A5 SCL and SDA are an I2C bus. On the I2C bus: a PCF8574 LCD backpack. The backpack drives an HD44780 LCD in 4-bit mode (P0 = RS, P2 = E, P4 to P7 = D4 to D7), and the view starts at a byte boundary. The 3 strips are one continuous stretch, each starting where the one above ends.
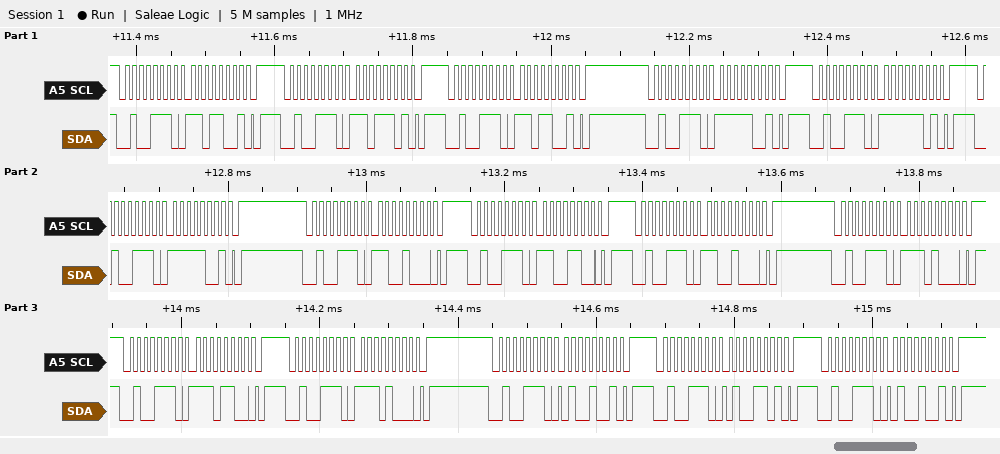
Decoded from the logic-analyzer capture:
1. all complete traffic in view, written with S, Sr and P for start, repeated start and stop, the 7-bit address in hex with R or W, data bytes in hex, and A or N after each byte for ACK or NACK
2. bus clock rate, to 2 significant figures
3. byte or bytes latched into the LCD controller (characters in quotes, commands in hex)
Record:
S 27W A D9 A P S 27W A DD A P S 27W A D9 A P S 27W A F9 A P S 27W A FD A P S 27W A F9 A P S 27W A C8 A P S 27W A CC A P S 27W A C8 A P S 27W A E8 A P S 27W A EC A P S 27W A E8 A P S 27W A 49 A P S 27W A 4D A P S 27W A 49 A P
100 kHz
data 0xDF 0xCE
